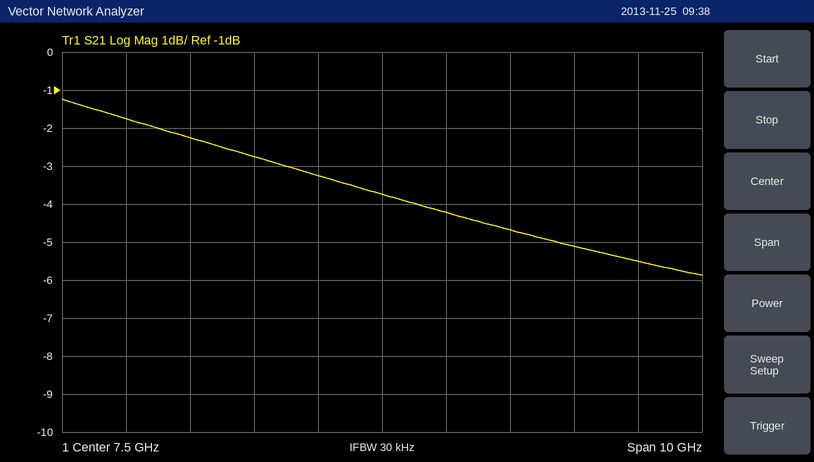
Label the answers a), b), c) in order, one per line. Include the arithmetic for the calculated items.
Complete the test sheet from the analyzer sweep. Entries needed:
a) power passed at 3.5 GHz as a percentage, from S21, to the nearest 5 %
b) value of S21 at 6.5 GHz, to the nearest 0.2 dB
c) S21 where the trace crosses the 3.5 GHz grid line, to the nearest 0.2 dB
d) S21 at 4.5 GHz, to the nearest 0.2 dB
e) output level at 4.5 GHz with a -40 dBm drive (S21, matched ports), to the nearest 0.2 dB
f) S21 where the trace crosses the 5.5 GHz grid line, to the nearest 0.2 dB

a) 10^(-1.8/10) ≈ 66.1 %, so 65 % to the nearest 5 %
b) -3.2 dB
c) -1.8 dB
d) -2.2 dB
e) -40 dBm + (-2.2 dB) = -42.2 dBm
f) -2.8 dB
